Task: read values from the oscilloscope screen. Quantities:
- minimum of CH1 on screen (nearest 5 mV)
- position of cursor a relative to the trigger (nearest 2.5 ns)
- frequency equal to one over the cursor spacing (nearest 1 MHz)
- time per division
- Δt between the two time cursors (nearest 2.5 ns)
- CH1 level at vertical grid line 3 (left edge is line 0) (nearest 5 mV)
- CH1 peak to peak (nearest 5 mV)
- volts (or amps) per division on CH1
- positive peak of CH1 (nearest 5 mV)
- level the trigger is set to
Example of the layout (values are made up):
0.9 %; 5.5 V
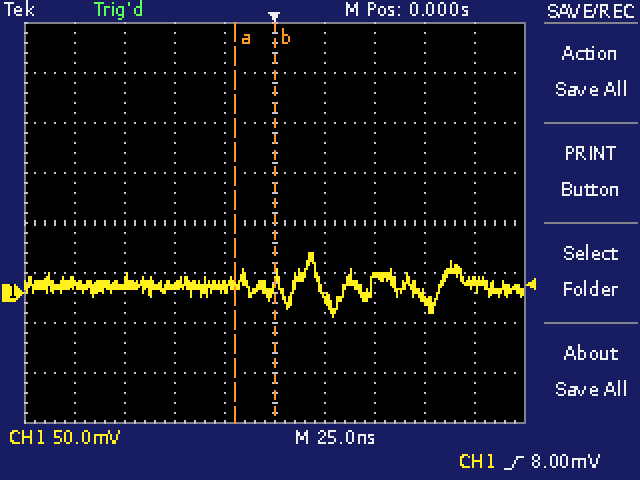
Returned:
-25 mV; -20.0 ns; 50 MHz; 25 ns; 20.0 ns; 10 mV; 65 mV; 50 mV; 40 mV; 8.00 mV
